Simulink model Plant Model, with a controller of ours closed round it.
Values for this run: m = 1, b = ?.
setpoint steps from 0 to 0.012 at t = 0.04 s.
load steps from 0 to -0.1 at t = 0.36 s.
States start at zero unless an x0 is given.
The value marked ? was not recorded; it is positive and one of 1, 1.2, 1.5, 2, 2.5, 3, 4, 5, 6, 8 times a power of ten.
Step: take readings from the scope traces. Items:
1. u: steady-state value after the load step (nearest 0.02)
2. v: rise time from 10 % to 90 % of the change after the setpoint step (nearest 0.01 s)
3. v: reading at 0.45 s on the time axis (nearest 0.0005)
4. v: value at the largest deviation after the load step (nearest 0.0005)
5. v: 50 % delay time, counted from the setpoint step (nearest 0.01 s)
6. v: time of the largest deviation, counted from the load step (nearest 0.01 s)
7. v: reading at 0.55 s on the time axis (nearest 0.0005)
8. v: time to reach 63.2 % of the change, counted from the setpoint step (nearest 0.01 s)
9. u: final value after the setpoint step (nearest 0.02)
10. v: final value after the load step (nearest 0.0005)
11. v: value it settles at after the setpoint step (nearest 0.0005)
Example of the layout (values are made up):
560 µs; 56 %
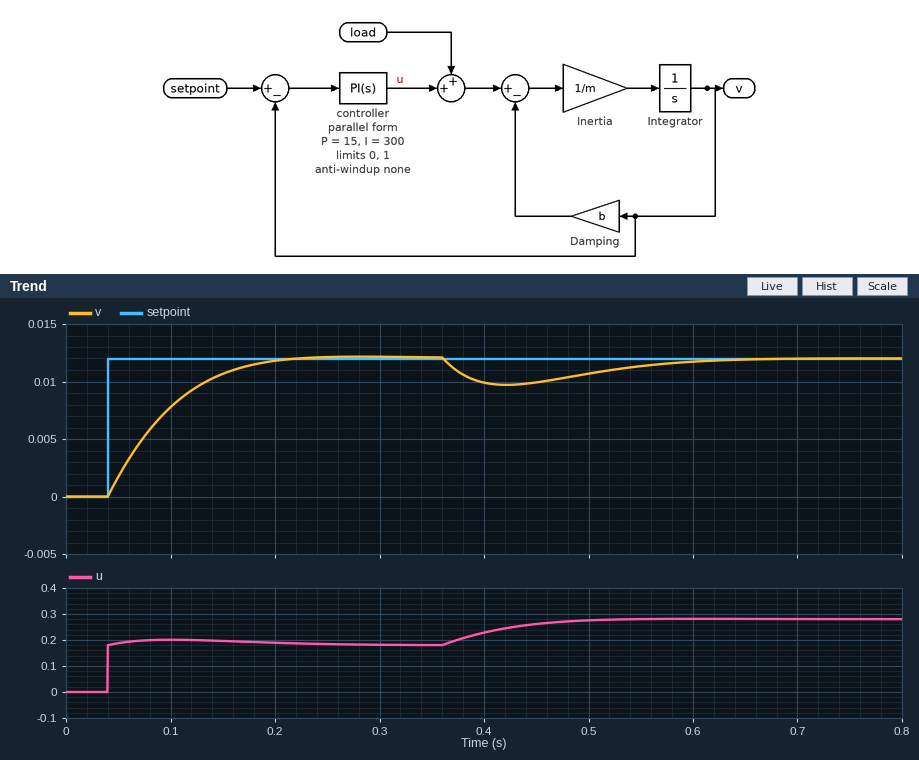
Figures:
0.28; 0.11 s; 0.0100; 0.0095; 0.04 s; 0.06 s; 0.0115; 0.06 s; 0.18; 0.0120; 0.0120
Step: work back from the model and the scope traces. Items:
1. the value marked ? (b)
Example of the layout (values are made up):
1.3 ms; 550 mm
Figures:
15
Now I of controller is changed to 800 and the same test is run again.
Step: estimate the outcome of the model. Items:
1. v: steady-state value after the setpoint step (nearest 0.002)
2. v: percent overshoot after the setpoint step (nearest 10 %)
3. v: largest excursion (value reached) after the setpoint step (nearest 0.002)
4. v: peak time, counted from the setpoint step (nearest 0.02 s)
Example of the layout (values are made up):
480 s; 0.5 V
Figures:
0.012; 20 %; 0.014; 0.10 s
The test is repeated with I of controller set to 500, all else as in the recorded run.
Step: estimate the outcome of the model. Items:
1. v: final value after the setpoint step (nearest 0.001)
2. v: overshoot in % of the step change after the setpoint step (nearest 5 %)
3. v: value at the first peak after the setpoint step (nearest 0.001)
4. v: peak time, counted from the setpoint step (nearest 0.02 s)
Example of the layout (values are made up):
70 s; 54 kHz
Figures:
0.012; 10 %; 0.013; 0.14 s
